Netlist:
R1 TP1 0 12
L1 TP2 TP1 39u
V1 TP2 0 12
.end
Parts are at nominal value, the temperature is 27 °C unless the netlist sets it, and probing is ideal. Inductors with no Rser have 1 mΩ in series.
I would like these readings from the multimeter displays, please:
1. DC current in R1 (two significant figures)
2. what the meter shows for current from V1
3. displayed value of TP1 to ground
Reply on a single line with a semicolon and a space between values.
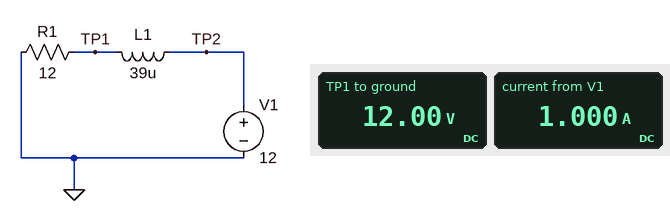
1.0 A; 1.000 A; 12.00 V
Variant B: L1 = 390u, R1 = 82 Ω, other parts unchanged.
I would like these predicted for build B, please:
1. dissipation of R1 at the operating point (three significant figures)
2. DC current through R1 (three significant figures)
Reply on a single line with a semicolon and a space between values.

1.76 W; 146 mA
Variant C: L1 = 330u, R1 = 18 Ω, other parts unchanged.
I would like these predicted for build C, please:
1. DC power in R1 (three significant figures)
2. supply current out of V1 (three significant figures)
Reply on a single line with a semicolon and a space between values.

8.00 W; 667 mA
